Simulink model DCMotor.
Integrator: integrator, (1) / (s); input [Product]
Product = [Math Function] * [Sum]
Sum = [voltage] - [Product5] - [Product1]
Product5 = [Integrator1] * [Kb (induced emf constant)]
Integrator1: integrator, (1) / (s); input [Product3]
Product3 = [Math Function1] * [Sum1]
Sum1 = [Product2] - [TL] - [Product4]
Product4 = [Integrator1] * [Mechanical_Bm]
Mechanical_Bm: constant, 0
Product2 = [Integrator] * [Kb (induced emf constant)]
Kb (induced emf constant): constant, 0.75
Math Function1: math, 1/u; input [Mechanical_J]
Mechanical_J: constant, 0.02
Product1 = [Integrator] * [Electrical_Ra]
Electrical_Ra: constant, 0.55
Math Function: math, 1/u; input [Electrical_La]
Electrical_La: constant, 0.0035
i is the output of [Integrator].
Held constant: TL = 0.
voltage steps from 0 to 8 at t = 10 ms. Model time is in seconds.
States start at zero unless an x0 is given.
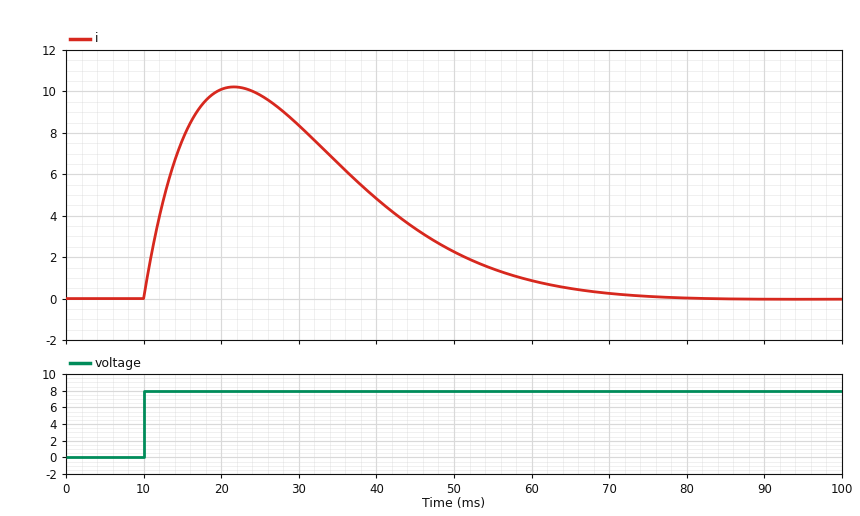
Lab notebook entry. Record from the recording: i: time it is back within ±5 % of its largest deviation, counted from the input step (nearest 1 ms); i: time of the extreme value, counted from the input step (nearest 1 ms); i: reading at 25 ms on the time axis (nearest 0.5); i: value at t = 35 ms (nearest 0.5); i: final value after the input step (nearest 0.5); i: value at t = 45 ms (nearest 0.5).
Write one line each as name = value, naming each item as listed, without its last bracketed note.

i: time it is back within ±5 % of its largest deviation, counted from the input step = 55 ms
i: time of the extreme value, counted from the input step = 12 ms
i: reading at 25 ms on the time axis = 10.0
i: value at t = 35 ms = 6.5
i: final value after the input step = 0.0
i: value at t = 45 ms = 3.5
